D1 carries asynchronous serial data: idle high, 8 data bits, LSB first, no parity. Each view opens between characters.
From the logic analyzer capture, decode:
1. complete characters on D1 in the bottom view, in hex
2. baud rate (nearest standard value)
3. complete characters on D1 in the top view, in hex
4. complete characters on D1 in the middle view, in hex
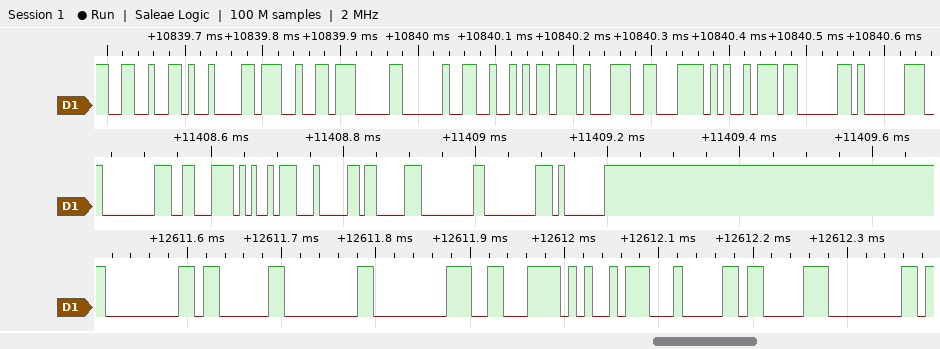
00, 03, 00, 00, C6, A5, 04, 83, 00
115200 baud
26, 09, 27, 07, 20, 52, 17, C6, A5, 03, 81
00, C6, A5, 04, 83, 00, 00, 01
